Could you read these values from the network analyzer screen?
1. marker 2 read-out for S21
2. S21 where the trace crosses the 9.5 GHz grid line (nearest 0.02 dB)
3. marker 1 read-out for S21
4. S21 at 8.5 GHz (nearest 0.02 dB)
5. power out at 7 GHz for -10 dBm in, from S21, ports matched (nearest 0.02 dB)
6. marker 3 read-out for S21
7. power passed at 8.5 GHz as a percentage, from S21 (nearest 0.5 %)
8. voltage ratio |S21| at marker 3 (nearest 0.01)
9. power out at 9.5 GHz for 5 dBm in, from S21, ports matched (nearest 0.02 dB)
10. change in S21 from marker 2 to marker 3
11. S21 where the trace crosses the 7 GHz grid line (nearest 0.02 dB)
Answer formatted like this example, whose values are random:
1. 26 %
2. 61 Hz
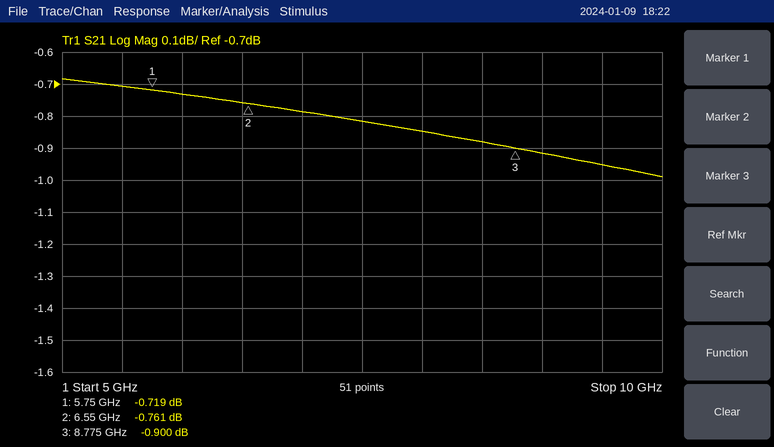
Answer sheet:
1. -0.761 dB
2. -0.96 dB
3. -0.719 dB
4. -0.88 dB
5. -10.78 dBm
6. -0.900 dB
7. 81.5 %
8. 0.90
9. 4.04 dBm
10. -0.139 dB
11. -0.78 dB
